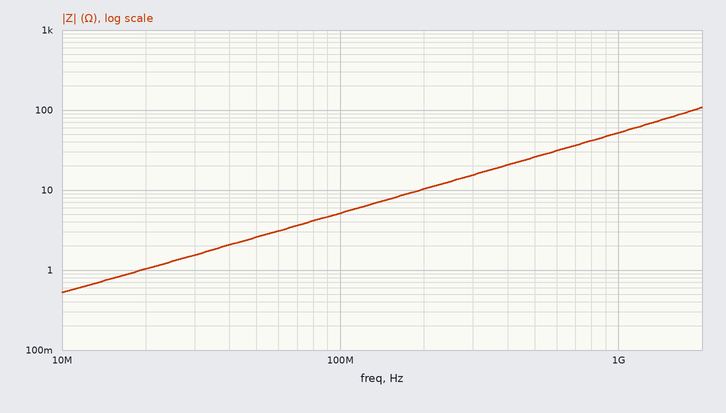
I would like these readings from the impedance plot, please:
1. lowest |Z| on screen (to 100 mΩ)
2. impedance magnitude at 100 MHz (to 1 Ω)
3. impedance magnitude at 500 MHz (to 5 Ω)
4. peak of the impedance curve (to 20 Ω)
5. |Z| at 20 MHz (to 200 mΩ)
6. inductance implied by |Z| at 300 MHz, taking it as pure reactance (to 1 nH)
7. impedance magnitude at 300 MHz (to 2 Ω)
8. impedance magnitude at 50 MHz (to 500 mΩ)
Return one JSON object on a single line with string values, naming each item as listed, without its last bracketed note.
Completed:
{"lowest |Z| on screen": "500 mΩ", "impedance magnitude at 100 MHz": "5 Ω", "impedance magnitude at 500 MHz": "25 Ω", "peak of the impedance curve": "100 Ω", "|Z| at 20 MHz": "1.0 Ω", "inductance implied by |Z| at 300 MHz, taking it as pure reactance": "8 nH", "impedance magnitude at 300 MHz": "16 Ω", "impedance magnitude at 50 MHz": "2.5 Ω"}
